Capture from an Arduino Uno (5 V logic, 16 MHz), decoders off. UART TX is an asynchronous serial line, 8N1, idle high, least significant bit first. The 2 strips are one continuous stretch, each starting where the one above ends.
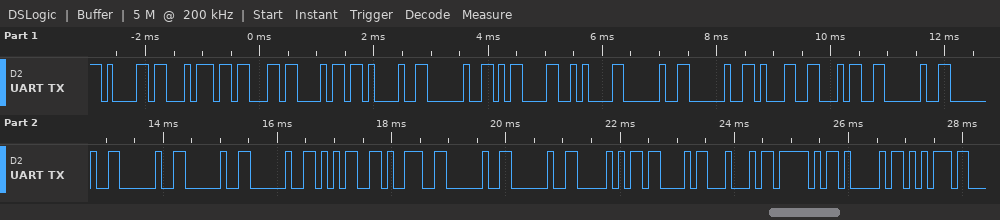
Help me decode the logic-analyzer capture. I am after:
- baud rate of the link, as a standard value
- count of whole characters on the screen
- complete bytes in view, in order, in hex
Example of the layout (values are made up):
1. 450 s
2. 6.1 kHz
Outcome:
1. 9600 baud
2. 27
3. 61 74 63 68 21 20 0D 0A 20 20 31 34 20 20 20 20 20 35 39 20 20 50 43 44 5F 41 75
